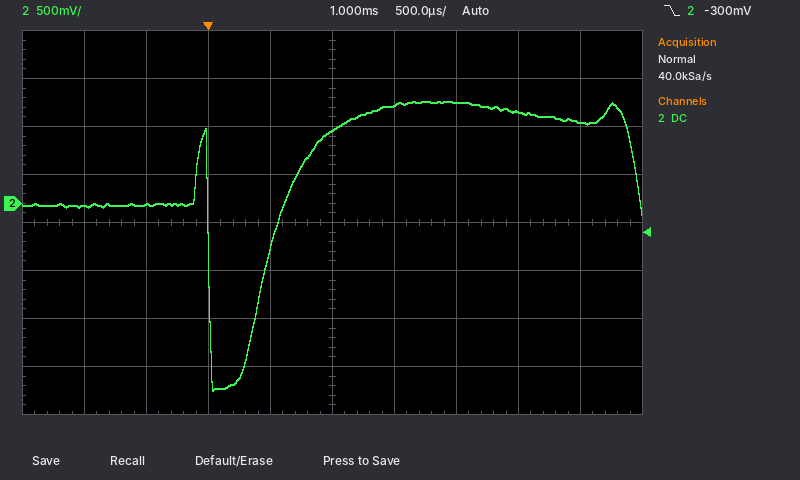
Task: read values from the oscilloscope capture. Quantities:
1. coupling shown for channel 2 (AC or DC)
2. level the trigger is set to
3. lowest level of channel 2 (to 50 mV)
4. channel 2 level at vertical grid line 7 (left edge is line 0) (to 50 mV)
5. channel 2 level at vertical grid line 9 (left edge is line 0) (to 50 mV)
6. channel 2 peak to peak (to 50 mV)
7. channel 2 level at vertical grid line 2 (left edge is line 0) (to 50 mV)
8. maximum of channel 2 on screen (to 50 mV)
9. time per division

DC
-300 mV
-1.95 V
1.05 V
850 mV
3.00 V
0 mV
1.05 V
500 µs
